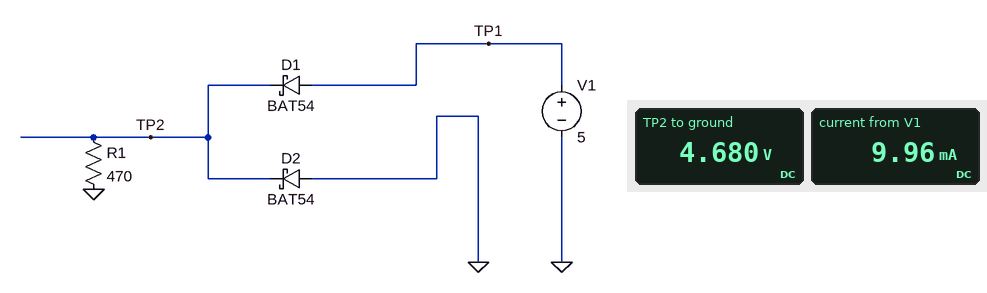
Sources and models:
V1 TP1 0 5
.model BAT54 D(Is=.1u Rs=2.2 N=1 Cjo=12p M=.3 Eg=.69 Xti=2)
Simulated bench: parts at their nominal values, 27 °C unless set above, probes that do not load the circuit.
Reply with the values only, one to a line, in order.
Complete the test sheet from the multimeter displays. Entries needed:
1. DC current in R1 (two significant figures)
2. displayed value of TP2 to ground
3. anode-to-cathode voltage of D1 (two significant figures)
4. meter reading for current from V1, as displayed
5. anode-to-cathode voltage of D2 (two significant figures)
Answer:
10 mA
4.680 V
320 mV
9.96 mA
-4.7 V
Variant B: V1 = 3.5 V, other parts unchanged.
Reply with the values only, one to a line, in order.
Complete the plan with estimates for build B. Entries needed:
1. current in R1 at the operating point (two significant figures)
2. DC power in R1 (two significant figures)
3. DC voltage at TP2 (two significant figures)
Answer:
6.8 mA
22 mW
3.2 V
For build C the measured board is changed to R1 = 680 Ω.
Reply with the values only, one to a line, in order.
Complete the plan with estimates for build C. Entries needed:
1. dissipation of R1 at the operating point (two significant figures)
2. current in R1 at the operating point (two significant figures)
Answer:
32 mW
6.9 mA
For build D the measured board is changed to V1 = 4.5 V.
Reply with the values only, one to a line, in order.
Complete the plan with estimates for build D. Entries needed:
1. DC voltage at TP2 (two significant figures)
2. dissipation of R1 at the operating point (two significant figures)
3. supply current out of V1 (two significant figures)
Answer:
4.2 V
37 mW
8.9 mA
